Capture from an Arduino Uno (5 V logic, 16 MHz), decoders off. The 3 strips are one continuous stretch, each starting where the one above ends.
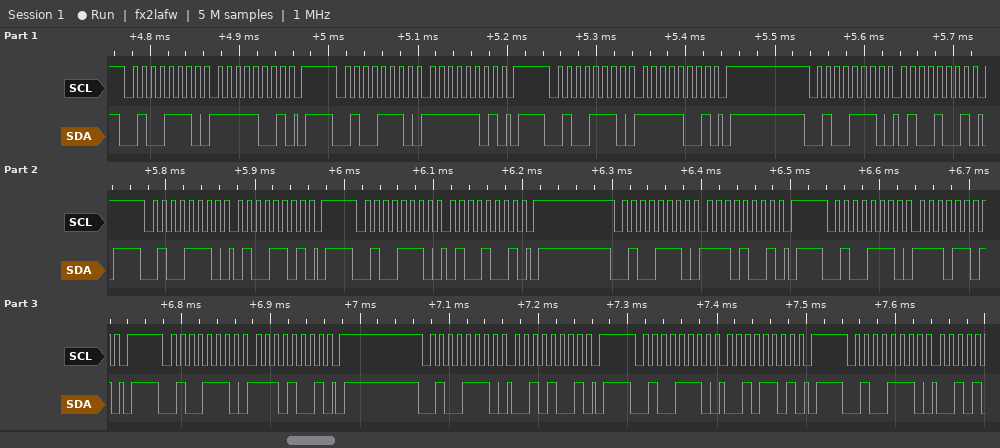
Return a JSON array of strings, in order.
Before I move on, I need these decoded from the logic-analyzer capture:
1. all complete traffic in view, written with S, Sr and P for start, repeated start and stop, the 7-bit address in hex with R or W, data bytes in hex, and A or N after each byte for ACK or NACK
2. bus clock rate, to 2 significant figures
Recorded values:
["S 27W A F9 A P S 27W A FD A P S 27W A F9 A P S 27W A 49 A P S 27W A 4D A P S 27W A 49 A P S 27W A E9 A P S 27W A ED A P S 27W A E9 A P S 27W A 29 A P S 27W A 2D A P S 27W A", "100 kHz"]
